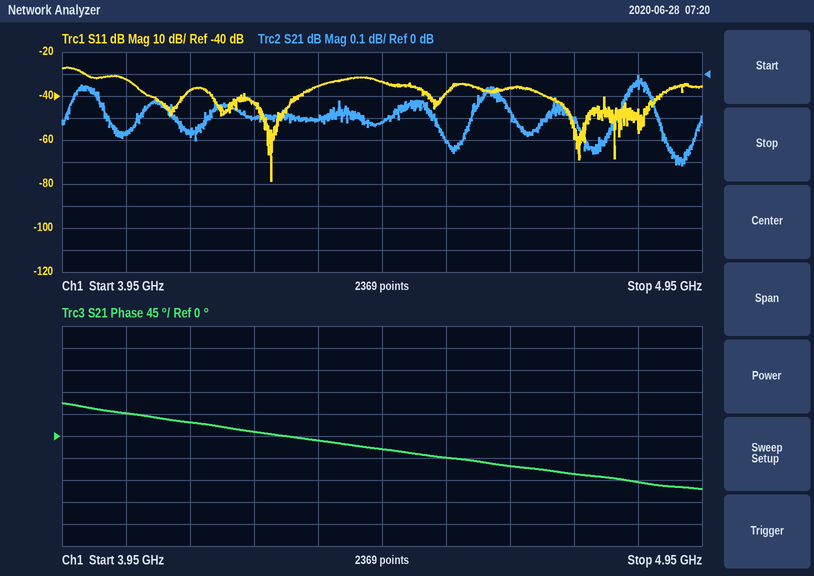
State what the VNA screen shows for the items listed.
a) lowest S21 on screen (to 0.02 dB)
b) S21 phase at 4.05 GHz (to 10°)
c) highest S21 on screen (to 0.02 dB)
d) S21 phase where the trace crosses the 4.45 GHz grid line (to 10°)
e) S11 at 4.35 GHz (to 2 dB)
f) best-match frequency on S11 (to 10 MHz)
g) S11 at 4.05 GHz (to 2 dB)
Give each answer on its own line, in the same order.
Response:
-0.42 dB
50°
0.00 dB
-30°
-36 dB
4.28 GHz
-32 dB
